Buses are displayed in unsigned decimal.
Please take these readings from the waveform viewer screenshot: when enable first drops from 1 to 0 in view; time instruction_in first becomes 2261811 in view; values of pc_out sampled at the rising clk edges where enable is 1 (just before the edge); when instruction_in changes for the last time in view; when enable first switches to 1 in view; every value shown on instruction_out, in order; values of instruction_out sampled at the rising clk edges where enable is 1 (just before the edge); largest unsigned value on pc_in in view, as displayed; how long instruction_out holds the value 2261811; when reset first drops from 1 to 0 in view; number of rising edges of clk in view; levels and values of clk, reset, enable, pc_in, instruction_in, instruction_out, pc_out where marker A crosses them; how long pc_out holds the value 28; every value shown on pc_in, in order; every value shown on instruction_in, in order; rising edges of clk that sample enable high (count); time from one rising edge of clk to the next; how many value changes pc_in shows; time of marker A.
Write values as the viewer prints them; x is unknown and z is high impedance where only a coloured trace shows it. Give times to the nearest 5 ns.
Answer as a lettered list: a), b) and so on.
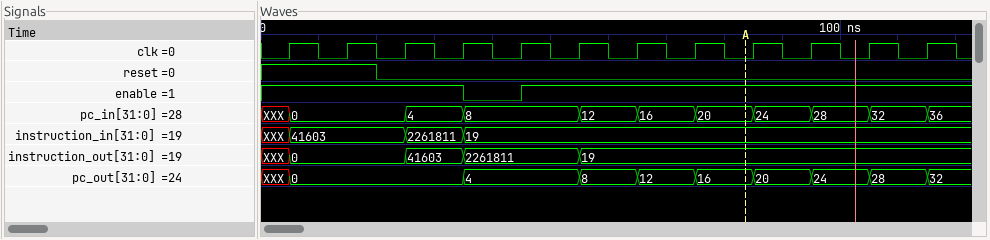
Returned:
a) 35 ns
b) 25 ns
c) XXX, 0, 0, 0, 4, 8, 12, 16, 20, 24, 28
d) 35 ns
e) 45 ns
f) XXX, 0, 41603, 2261811, 19
g) XXX, 0, 0, 41603, 2261811, 19, 19, 19, 19, 19, 19
h) 36
i) 20 ns
j) 20 ns
k) 12
l) clk=0, reset=0, enable=1, pc_in=20, instruction_in=19, instruction_out=19, pc_out=16
m) 10 ns
n) XXX, 0, 4, 8, 12, 16, 20, 24, 28, 32, 36
o) XXX, 41603, 2261811, 19
p) 11
q) 10 ns
r) 10
s) 85 ns
